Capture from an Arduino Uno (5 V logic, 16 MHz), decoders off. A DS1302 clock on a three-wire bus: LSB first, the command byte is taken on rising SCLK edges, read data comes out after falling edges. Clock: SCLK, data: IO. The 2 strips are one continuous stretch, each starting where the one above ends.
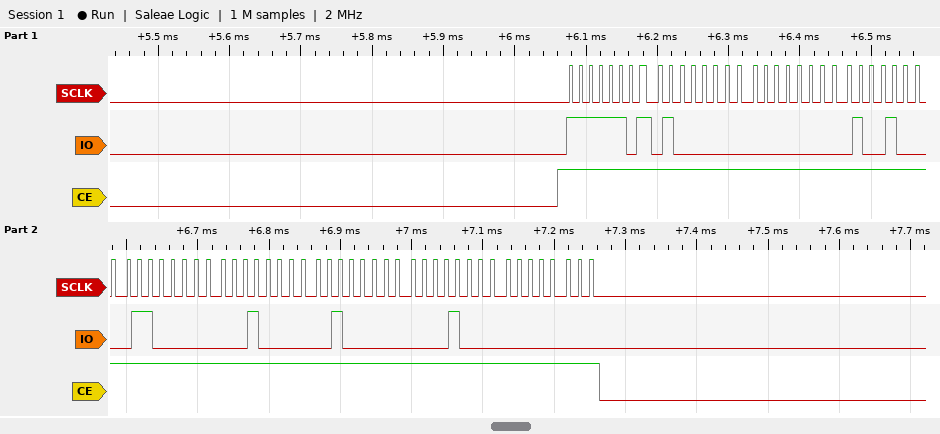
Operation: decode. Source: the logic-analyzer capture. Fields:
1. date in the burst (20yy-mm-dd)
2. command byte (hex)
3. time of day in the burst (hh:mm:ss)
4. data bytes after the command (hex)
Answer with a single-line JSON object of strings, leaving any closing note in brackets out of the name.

{"date in the burst": "2010-08-06", "command byte": "0xBF", "time of day in the burst": "12:00:02", "data bytes after the command": "02 00 12 06 08 04 10 00"}
